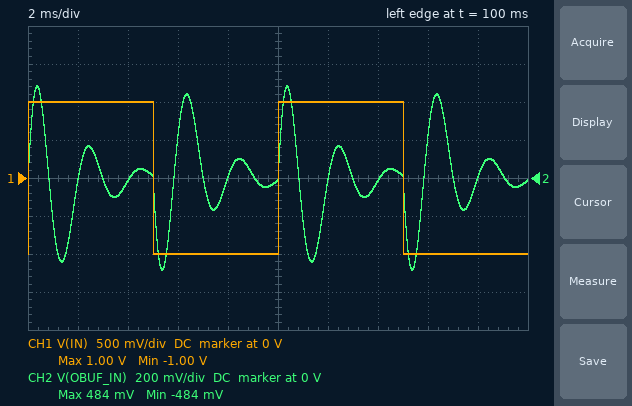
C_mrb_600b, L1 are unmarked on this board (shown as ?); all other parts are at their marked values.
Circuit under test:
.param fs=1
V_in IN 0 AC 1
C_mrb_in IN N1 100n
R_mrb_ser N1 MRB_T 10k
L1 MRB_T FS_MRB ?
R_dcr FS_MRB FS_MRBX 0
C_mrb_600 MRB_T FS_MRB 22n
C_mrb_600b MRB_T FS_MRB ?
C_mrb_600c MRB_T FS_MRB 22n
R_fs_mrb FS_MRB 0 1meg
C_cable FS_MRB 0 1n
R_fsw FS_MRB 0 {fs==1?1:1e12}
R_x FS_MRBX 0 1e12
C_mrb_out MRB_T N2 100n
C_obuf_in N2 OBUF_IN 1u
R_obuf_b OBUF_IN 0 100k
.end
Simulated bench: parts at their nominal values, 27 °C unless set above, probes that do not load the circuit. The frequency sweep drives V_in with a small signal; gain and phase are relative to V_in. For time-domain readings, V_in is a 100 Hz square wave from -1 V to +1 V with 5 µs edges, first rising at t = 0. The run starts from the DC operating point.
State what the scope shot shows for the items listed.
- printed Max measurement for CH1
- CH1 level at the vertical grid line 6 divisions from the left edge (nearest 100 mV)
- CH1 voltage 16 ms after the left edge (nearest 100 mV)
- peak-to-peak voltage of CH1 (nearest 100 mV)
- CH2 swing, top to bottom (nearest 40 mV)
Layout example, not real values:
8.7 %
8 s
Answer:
1.00 V
1.0 V
-1.0 V
2.0 V
960 mV
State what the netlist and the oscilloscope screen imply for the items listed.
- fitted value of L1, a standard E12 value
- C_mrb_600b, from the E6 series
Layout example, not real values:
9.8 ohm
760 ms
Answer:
1.2 H
33 nF
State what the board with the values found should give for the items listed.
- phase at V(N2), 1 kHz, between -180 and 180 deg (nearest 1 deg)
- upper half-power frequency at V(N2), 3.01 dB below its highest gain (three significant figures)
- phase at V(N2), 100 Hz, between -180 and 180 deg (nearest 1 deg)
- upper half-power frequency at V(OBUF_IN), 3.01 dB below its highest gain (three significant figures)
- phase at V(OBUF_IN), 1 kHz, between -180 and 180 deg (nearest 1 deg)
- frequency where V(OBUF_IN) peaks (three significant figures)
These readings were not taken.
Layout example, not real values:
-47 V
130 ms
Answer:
-64 deg
608 Hz
155 deg
608 Hz
-64 deg
492 Hz
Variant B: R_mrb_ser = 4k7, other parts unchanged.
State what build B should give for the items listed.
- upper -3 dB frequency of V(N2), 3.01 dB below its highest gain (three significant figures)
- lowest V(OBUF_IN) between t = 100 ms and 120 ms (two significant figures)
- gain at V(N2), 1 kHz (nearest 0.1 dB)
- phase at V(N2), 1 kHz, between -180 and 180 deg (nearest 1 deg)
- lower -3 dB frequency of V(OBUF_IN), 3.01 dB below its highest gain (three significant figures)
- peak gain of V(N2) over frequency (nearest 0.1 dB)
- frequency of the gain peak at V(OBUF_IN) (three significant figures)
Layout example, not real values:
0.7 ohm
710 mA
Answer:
572 Hz
-640 mV
-7.2 dB
-45 deg
330 Hz
1.5 dB
416 Hz
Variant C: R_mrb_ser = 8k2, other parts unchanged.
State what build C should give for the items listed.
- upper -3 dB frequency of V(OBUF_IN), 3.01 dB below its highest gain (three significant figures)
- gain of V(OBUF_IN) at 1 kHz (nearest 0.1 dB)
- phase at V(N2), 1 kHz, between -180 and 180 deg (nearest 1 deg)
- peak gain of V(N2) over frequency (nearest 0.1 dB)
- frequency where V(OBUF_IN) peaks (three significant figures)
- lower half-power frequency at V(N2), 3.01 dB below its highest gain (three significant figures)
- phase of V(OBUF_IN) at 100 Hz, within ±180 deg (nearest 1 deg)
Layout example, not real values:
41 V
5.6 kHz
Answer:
613 Hz
-10.4 dB
-59 deg
-0.1 dB
478 Hz
381 Hz
161 deg
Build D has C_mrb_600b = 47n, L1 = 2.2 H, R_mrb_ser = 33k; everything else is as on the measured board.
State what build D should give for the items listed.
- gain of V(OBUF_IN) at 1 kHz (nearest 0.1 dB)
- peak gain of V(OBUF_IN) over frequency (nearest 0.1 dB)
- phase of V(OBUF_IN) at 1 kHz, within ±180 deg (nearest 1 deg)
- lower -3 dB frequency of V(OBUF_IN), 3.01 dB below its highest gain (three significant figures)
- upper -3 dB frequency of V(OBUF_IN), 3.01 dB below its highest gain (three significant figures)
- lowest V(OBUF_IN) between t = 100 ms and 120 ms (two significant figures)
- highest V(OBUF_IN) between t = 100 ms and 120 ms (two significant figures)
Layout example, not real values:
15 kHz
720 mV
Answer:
-24.4 dB
-2.4 dB
-82 deg
319 Hz
388 Hz
-220 mV
220 mV
